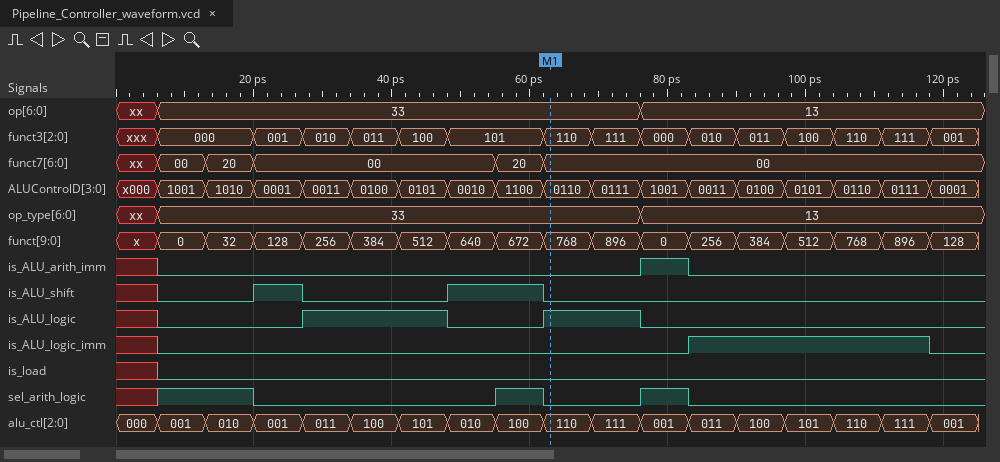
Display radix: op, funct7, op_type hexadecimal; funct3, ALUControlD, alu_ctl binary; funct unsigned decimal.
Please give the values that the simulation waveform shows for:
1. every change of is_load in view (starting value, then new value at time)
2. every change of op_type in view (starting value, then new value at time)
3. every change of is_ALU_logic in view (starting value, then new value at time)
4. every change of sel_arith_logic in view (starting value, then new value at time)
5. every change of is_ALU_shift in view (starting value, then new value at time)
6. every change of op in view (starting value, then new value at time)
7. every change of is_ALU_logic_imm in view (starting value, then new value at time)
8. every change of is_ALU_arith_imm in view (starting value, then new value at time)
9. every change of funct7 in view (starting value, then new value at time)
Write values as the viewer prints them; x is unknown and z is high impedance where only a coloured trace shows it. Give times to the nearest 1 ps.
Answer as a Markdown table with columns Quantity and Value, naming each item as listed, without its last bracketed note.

| Quantity | Value |
|---|---|
| every change of is_load in view | x, 0 at 6 ps |
| every change of op_type in view | xx, 33 at 6 ps, 13 at 76 ps |
| every change of is_ALU_logic in view | x, 0 at 6 ps, 1 at 27 ps, 0 at 48 ps, 1 at 62 ps, 0 at 76 ps |
| every change of sel_arith_logic in view | x, 1 at 6 ps, 0 at 20 ps, 1 at 55 ps, 0 at 62 ps, 1 at 76 ps, 0 at 83 ps |
| every change of is_ALU_shift in view | x, 0 at 6 ps, 1 at 20 ps, 0 at 27 ps, 1 at 48 ps, 0 at 62 ps |
| every change of op in view | xx, 33 at 6 ps, 13 at 76 ps |
| every change of is_ALU_logic_imm in view | x, 0 at 6 ps, 1 at 83 ps, 0 at 118 ps |
| every change of is_ALU_arith_imm in view | x, 0 at 6 ps, 1 at 76 ps, 0 at 83 ps |
| every change of funct7 in view | xx, 00 at 6 ps, 20 at 13 ps, 00 at 20 ps, 20 at 55 ps, 00 at 62 ps |
